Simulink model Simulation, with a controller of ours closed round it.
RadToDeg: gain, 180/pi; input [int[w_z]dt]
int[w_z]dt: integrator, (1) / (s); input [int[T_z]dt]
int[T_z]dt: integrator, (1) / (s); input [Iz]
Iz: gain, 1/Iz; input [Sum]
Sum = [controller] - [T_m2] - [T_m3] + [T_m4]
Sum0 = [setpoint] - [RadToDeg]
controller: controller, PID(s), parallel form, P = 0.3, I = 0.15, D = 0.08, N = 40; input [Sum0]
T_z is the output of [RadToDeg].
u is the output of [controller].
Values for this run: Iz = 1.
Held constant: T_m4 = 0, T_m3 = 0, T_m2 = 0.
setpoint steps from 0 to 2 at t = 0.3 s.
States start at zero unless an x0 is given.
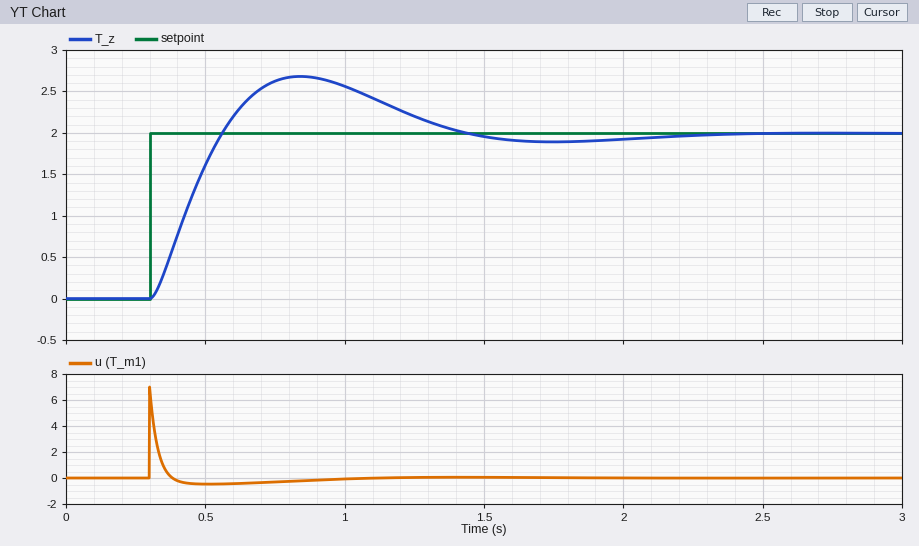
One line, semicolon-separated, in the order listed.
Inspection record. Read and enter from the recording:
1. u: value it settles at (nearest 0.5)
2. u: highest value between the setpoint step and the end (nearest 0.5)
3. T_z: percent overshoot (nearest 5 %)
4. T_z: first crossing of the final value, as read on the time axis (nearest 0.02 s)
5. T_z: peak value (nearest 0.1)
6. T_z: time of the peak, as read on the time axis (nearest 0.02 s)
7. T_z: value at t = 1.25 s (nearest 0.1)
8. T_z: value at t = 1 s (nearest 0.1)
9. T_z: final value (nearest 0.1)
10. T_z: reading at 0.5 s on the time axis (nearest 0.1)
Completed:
0.0; 7.0; 35 %; 0.56 s; 2.7; 0.84 s; 2.2; 2.6; 2.0; 1.6
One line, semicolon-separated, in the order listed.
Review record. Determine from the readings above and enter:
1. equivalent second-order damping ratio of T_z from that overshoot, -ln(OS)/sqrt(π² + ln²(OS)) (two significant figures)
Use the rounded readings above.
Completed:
0.32
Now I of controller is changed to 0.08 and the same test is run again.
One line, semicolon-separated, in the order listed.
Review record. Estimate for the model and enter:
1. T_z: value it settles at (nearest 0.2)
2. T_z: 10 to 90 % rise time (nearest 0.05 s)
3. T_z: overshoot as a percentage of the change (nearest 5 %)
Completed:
2.0; 0.20 s; 30 %
